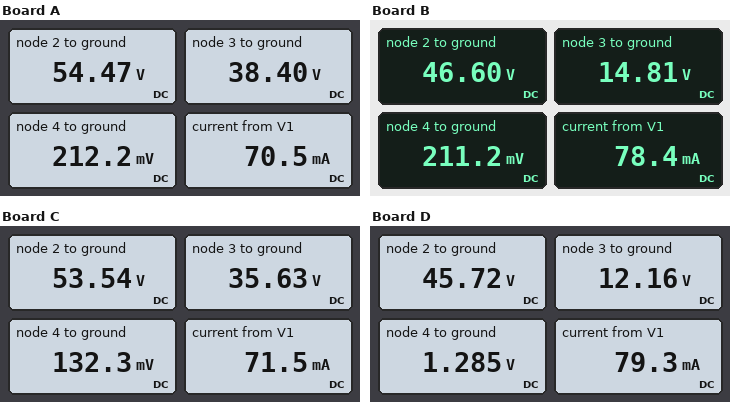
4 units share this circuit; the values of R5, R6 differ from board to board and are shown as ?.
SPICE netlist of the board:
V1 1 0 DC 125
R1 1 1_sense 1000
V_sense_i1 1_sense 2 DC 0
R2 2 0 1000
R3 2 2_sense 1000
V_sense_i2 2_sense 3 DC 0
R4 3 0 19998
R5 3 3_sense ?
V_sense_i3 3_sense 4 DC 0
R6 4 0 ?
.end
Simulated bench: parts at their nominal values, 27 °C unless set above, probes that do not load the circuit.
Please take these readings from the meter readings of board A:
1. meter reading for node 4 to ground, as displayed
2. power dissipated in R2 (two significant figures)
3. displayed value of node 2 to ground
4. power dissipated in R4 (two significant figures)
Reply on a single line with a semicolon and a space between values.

212.2 mV; 3.0 W; 54.47 V; 74 mW
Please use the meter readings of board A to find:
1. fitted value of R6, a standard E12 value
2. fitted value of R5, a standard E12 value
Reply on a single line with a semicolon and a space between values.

15 Ω; 2.7 kΩ
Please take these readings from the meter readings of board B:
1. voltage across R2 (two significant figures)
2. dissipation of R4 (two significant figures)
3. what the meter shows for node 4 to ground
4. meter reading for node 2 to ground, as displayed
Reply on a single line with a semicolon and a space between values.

47 V; 11 mW; 211.2 mV; 46.60 V
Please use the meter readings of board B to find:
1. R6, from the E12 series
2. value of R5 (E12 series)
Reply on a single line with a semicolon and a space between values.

6.8 Ω; 470 Ω
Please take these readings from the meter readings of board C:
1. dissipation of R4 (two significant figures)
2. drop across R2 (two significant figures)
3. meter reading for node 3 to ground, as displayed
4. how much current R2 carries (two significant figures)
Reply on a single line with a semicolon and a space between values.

63 mW; 54 V; 35.63 V; 54 mA
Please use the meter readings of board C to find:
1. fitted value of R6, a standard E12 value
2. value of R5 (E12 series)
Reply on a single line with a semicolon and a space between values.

8.2 Ω; 2.2 kΩ
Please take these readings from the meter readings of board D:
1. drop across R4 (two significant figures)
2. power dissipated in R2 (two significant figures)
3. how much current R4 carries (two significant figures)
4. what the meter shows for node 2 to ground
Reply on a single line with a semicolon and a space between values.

12 V; 2.1 W; 610 µA; 45.72 V
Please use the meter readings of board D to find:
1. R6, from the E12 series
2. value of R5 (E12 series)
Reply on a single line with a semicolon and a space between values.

39 Ω; 330 Ω
